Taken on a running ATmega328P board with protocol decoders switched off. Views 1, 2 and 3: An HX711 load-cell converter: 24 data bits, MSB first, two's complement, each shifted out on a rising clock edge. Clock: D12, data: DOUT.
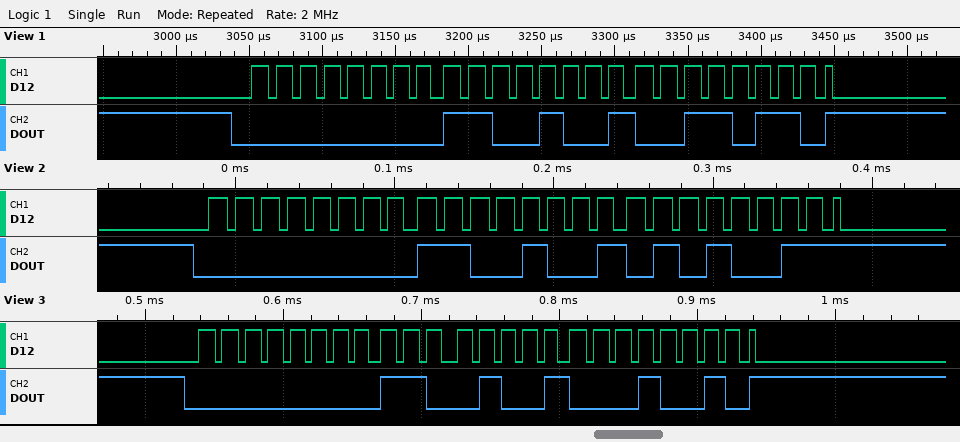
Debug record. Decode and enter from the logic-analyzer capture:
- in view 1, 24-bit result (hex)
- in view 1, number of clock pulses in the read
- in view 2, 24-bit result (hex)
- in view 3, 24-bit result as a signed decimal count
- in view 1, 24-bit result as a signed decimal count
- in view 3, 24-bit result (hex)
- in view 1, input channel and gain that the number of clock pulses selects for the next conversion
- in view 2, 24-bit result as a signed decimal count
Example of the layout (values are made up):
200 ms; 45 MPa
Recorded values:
0x00C936; 25; 0x00C953; 51474; 51510; 0x00C912; channel A, gain 128; 51539
